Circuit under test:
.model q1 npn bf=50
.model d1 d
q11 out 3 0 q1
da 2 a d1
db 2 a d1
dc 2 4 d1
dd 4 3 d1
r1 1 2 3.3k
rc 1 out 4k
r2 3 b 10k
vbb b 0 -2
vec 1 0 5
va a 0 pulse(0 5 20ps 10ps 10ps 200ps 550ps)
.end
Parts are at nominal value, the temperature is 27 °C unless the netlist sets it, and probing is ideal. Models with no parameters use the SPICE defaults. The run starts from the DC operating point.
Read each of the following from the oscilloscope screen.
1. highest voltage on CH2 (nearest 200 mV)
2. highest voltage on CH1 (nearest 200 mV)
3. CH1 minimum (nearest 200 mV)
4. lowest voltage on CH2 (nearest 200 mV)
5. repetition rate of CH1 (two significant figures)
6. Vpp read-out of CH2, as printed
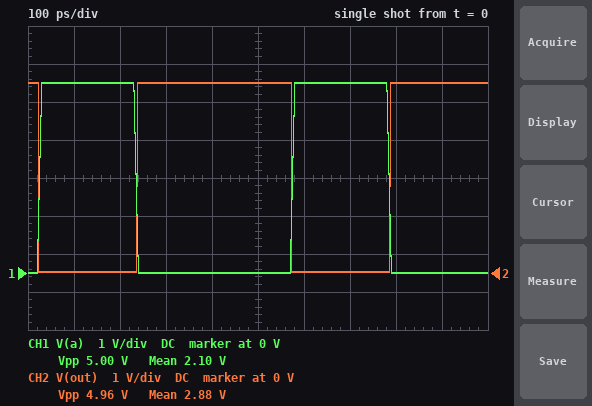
5.0 V
5.0 V
0 V
0 V
1.8 GHz
4.96 V
